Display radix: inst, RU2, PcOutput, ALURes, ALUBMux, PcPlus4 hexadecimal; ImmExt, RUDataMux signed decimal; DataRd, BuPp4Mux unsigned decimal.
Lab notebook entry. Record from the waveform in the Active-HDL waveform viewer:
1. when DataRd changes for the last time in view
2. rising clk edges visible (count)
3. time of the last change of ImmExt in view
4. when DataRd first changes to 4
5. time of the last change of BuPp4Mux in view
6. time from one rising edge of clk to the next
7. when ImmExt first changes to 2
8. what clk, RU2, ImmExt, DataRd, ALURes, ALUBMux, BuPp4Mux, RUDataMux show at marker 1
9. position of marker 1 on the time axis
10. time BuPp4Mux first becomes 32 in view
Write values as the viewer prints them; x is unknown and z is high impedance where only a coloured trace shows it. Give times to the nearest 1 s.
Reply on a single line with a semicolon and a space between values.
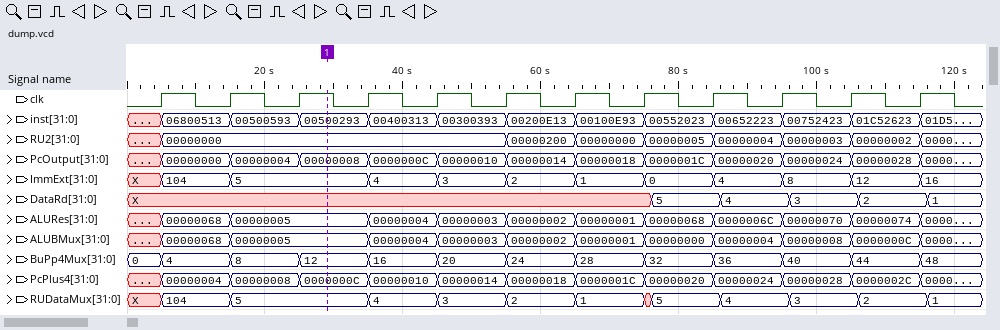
116 s; 12; 115 s; 86 s; 115 s; 10 s; 55 s; clk=1, RU2=00000000, ImmExt=5, DataRd=X, ALURes=00000005, ALUBMux=00000005, BuPp4Mux=12, RUDataMux=5; 29 s; 75 s
